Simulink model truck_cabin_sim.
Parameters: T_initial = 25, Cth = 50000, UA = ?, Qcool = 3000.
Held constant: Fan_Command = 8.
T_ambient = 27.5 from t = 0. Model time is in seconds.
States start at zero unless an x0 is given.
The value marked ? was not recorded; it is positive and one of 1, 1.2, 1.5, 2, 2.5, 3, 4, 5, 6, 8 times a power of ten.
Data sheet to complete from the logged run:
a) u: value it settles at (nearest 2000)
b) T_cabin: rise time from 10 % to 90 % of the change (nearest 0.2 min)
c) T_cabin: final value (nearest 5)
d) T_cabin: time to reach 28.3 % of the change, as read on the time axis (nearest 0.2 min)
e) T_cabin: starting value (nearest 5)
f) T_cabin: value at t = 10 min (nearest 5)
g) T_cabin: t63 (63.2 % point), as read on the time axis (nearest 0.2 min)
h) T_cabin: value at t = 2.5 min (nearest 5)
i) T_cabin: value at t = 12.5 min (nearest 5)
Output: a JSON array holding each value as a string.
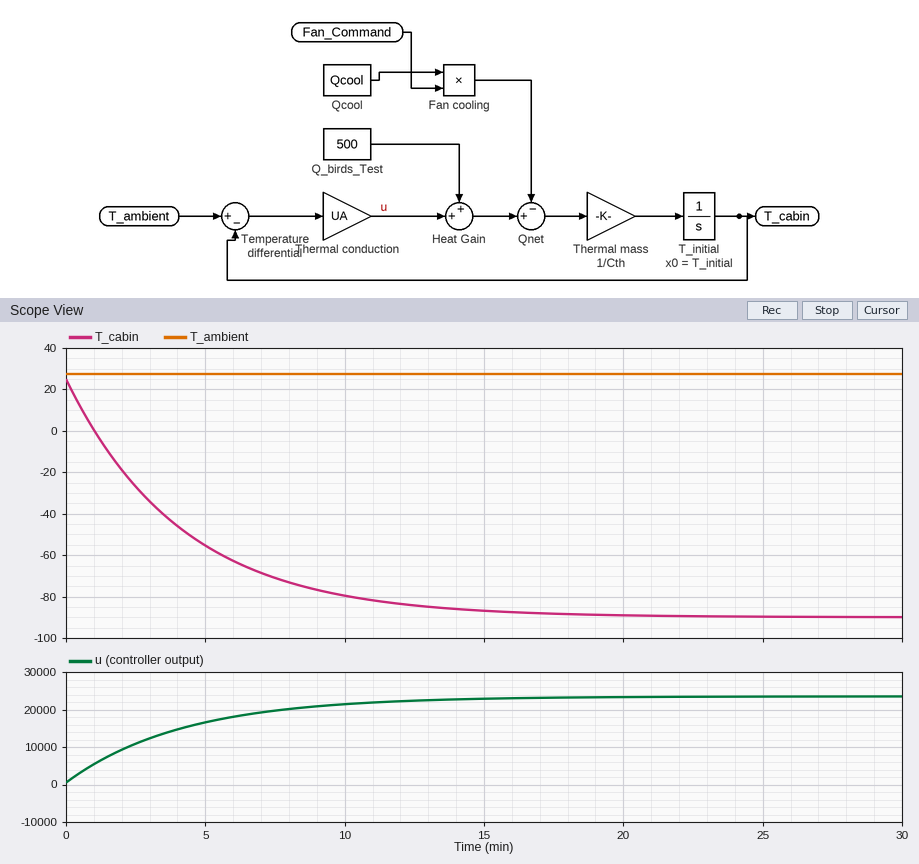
["24000", "9.2 min", "-90", "1.4 min", "25", "-80", "4.2 min", "-25", "-85"]
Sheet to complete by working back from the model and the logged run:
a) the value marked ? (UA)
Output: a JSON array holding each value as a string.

["200"]
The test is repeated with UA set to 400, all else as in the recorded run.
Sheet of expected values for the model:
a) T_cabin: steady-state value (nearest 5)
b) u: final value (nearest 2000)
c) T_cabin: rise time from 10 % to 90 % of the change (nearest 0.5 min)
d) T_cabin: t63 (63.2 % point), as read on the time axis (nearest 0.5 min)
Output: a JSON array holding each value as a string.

["-30", "24000", "4.5 min", "2.0 min"]
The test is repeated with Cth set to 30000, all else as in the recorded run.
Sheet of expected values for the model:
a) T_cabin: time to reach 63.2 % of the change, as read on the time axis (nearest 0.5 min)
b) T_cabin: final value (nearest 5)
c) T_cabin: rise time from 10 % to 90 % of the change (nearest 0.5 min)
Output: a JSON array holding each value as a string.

["2.5 min", "-90", "5.5 min"]
